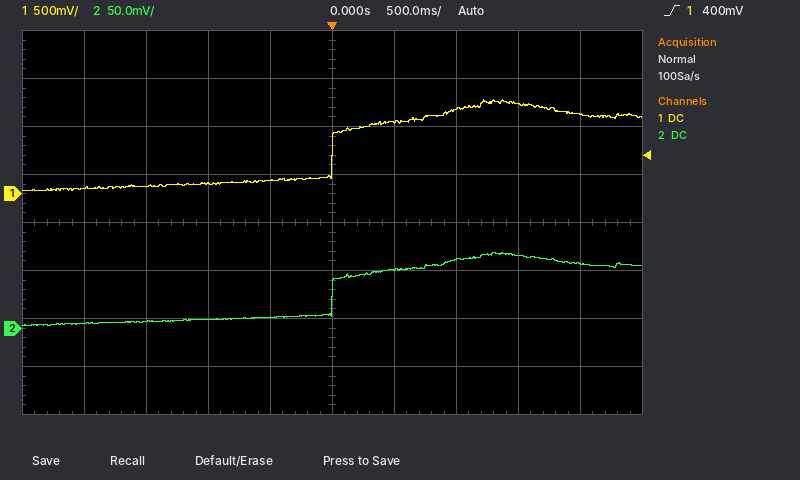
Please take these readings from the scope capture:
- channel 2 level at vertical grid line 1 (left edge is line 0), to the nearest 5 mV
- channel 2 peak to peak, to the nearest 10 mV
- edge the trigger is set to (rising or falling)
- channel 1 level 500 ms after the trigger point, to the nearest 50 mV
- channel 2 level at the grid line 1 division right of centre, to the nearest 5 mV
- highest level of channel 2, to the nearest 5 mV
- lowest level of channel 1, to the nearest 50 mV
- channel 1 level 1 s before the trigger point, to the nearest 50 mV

5 mV
80 mV
rising
750 mV
60 mV
80 mV
50 mV
100 mV
